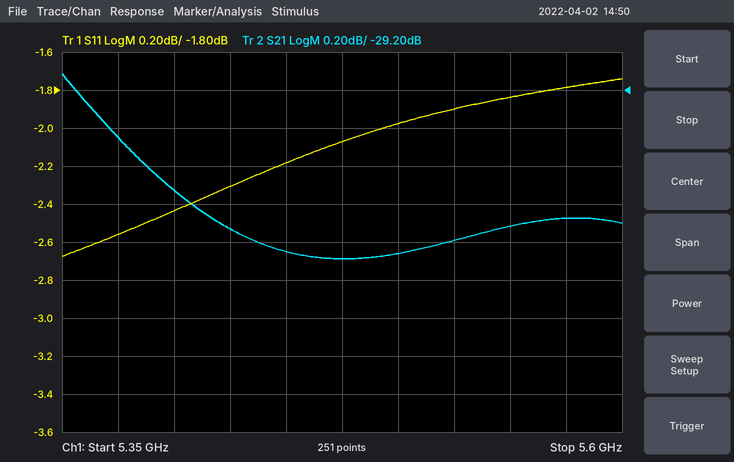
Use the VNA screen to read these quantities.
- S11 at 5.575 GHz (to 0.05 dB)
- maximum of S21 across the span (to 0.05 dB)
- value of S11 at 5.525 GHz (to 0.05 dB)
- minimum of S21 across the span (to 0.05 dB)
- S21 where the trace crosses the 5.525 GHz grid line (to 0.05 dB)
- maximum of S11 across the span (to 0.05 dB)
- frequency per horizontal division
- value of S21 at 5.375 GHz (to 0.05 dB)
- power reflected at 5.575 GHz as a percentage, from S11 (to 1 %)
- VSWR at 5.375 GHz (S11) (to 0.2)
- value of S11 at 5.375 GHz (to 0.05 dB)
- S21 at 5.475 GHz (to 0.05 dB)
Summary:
-1.80 dB
-29.10 dB
-1.90 dB
-30.10 dB
-30.00 dB
-1.75 dB
25 MHz
-29.45 dB
66 %
6.8
-2.55 dB
-30.10 dB
